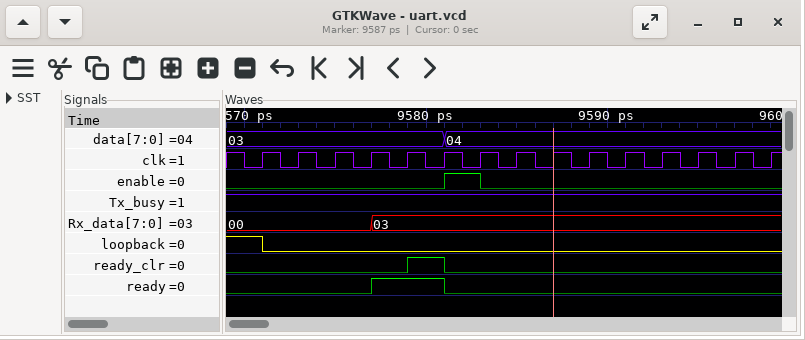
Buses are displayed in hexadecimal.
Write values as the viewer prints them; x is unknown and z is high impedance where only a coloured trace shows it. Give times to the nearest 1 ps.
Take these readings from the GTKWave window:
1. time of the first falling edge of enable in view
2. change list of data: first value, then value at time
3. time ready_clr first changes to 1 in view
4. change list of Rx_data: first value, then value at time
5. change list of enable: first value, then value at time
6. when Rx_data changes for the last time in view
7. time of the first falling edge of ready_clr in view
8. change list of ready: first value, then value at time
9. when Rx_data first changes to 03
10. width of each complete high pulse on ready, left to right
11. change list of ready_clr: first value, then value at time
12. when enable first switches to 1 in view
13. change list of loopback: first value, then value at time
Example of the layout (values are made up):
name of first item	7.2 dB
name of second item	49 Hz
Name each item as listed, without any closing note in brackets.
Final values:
time of the first falling edge of enable in view	9583 ps
change list of data: first value, then value at time	03, 04 at 9581 ps
time ready_clr first changes to 1 in view	9579 ps
change list of Rx_data: first value, then value at time	00, 03 at 9577 ps
change list of enable: first value, then value at time	0, 1 at 9581 ps, 0 at 9583 ps
when Rx_data changes for the last time in view	9577 ps
time of the first falling edge of ready_clr in view	9581 ps
change list of ready: first value, then value at time	0, 1 at 9577 ps, 0 at 9581 ps
when Rx_data first changes to 03	9577 ps
width of each complete high pulse on ready, left to right	4 ps
change list of ready_clr: first value, then value at time	0, 1 at 9579 ps, 0 at 9581 ps
when enable first switches to 1 in view	9581 ps
change list of loopback: first value, then value at time	1, 0 at 9571 ps
